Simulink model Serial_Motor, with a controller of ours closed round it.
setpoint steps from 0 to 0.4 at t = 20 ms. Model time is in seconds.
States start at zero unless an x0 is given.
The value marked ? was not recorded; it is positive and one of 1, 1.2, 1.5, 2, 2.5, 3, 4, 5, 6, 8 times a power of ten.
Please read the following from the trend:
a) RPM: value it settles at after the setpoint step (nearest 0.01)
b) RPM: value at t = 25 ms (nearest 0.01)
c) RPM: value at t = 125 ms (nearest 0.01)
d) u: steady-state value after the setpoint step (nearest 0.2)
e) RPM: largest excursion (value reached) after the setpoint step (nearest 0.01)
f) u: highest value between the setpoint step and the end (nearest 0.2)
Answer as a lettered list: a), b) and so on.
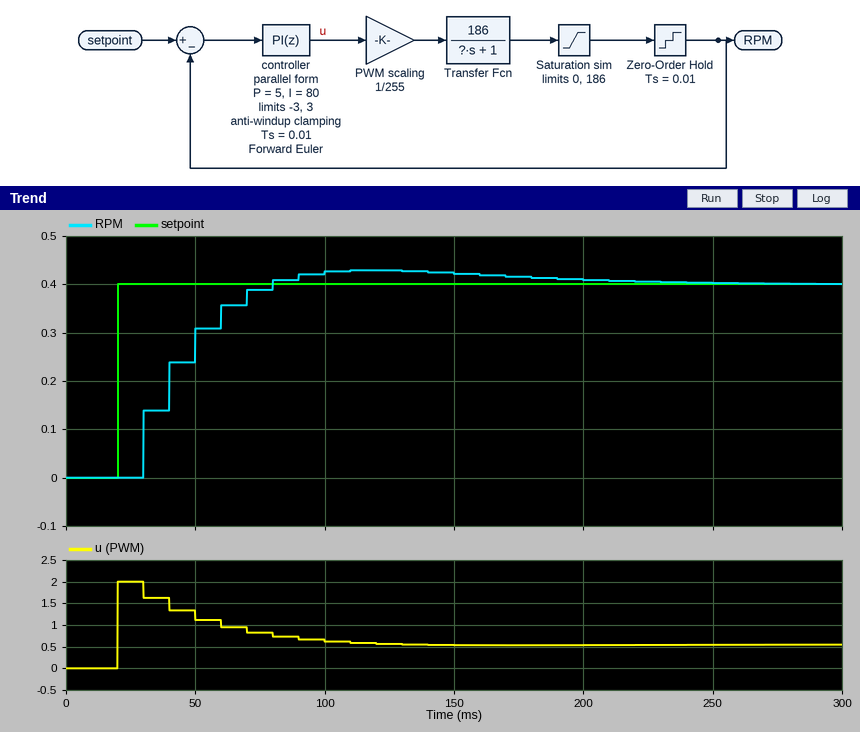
a) 0.40
b) 0.00
c) 0.43
d) 0.6
e) 0.43
f) 2.0
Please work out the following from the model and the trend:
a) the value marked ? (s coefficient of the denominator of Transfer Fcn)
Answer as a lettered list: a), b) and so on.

a) 0.1
